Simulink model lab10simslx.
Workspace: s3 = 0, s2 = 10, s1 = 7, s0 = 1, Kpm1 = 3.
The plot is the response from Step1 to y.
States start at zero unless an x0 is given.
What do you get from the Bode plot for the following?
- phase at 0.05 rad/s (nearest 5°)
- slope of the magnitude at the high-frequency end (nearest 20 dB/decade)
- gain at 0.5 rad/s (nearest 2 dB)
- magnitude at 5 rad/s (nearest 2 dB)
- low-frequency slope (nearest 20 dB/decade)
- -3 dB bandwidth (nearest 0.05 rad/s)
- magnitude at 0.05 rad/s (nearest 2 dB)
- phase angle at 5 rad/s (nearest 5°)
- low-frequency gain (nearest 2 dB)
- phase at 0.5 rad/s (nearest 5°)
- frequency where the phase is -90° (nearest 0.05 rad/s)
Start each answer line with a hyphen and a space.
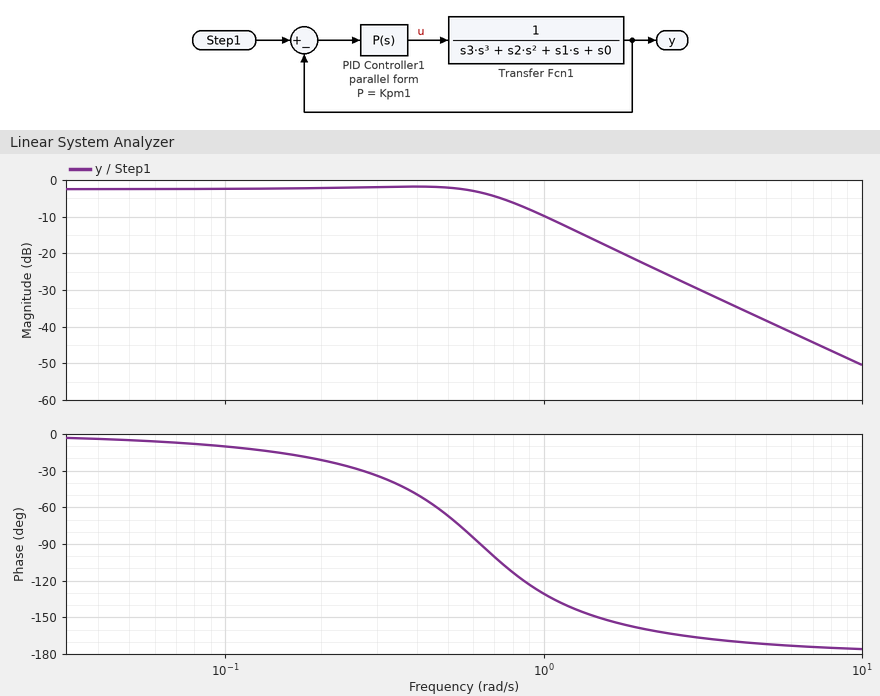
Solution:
- -5°
- -40 dB/decade
- -2 dB
- -38 dB
- 0 dB/decade
- 0.75 rad/s
- -2 dB
- -170°
- -2 dB
- -65°
- 0.65 rad/s
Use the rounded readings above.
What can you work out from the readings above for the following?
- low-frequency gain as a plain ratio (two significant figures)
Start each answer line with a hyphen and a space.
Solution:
- 0.79
